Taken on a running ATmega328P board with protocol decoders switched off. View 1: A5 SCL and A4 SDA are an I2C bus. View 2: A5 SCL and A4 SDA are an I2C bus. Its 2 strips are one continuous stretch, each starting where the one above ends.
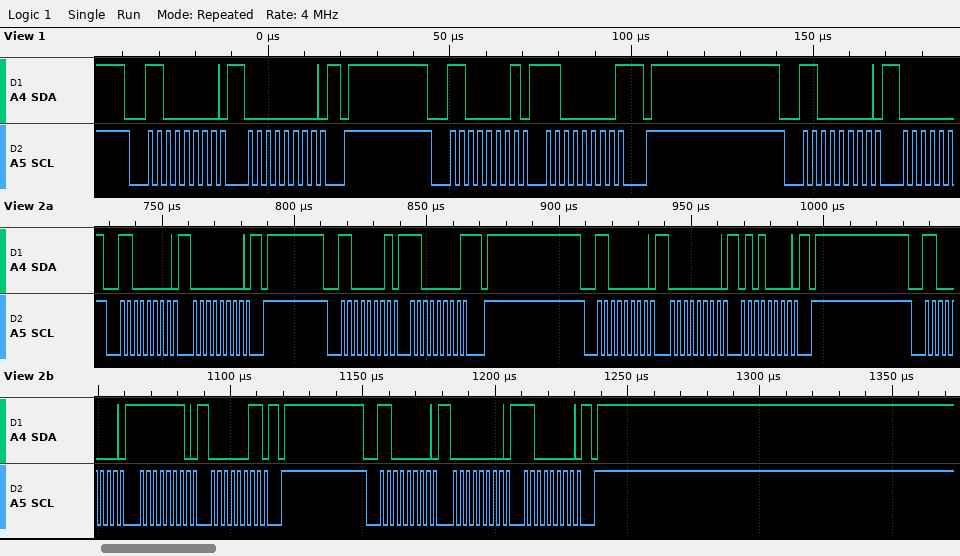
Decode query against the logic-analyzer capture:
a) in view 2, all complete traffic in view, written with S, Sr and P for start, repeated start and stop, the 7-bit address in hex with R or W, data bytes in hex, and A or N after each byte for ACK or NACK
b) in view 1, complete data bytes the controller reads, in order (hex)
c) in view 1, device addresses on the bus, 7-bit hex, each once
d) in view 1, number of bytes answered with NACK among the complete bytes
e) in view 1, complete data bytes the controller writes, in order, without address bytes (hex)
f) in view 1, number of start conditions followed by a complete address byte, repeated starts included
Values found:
S 60W A 00 A P S 60R A C0 N P S 60W A 00 A 50 A P S 60W A FE A 03 A P S 60W A 00 A C0 A P
C0
0x60
1
00
3
